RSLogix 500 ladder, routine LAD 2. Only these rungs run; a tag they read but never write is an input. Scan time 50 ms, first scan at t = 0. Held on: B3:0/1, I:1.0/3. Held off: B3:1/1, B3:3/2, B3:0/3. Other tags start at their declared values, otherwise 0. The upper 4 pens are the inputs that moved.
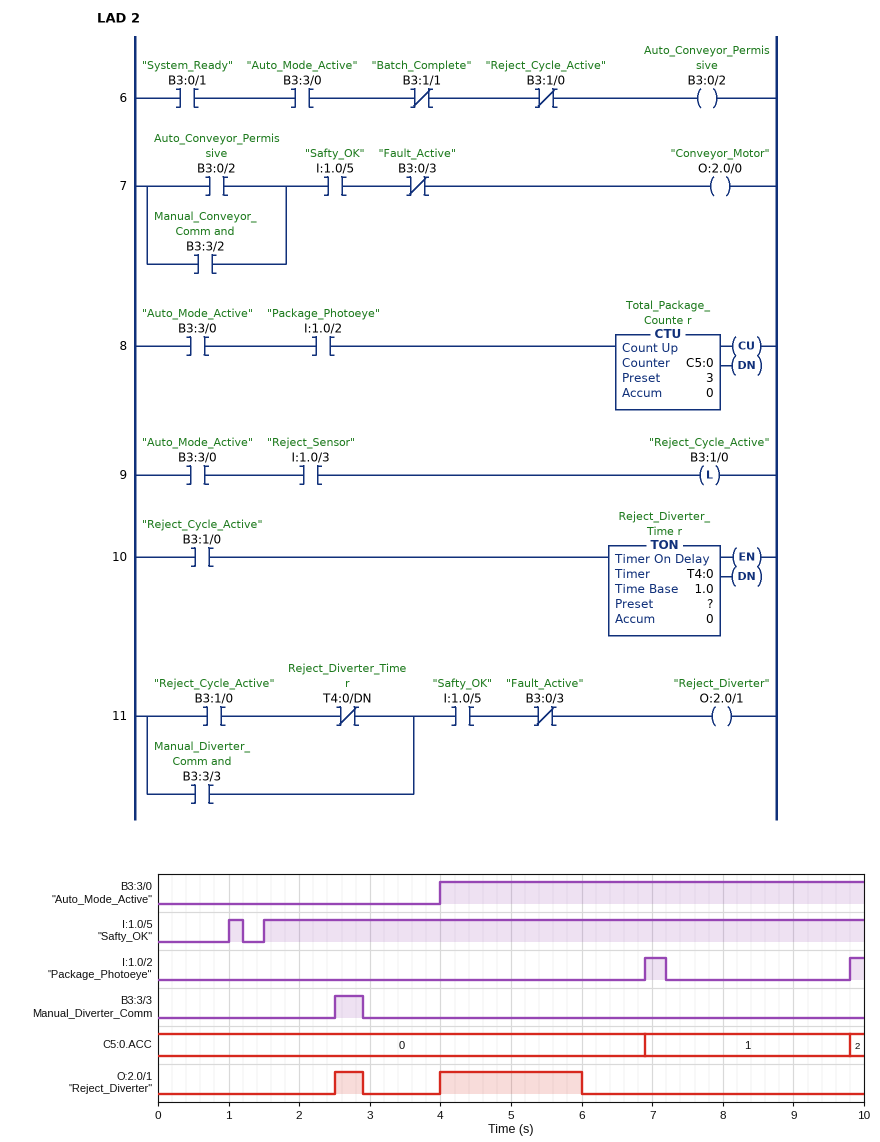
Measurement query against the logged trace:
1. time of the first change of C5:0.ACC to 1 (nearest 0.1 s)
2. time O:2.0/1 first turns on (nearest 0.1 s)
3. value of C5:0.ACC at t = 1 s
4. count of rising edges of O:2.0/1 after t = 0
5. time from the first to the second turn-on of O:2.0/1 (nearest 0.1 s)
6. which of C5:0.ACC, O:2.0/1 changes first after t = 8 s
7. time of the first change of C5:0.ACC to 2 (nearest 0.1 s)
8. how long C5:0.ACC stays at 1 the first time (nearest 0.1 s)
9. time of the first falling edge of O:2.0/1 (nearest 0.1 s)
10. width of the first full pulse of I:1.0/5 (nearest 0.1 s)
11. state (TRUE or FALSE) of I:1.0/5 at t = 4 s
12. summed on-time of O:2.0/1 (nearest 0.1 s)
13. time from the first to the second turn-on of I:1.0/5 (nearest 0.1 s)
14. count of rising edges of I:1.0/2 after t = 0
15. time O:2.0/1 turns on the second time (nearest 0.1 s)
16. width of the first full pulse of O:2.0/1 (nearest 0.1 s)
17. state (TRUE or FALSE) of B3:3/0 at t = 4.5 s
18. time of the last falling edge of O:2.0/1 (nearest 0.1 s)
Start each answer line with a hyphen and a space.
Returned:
- 6.9 s
- 2.5 s
- 0
- 2
- 1.5 s
- C5:0.ACC
- 9.8 s
- 2.9 s
- 2.9 s
- 0.2 s
- TRUE
- 2.4 s
- 0.5 s
- 2
- 4.0 s
- 0.4 s
- TRUE
- 6.0 s
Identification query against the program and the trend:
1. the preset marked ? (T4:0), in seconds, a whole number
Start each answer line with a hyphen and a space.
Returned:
- 2 s
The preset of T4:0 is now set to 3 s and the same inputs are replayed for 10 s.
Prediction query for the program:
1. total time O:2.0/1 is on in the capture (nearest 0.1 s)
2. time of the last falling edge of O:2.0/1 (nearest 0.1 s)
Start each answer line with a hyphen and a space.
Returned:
- 3.4 s
- 7.0 s
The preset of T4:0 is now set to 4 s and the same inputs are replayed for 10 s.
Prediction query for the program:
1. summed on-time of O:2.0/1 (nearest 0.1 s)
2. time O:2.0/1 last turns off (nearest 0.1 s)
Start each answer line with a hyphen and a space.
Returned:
- 4.4 s
- 8.0 s
